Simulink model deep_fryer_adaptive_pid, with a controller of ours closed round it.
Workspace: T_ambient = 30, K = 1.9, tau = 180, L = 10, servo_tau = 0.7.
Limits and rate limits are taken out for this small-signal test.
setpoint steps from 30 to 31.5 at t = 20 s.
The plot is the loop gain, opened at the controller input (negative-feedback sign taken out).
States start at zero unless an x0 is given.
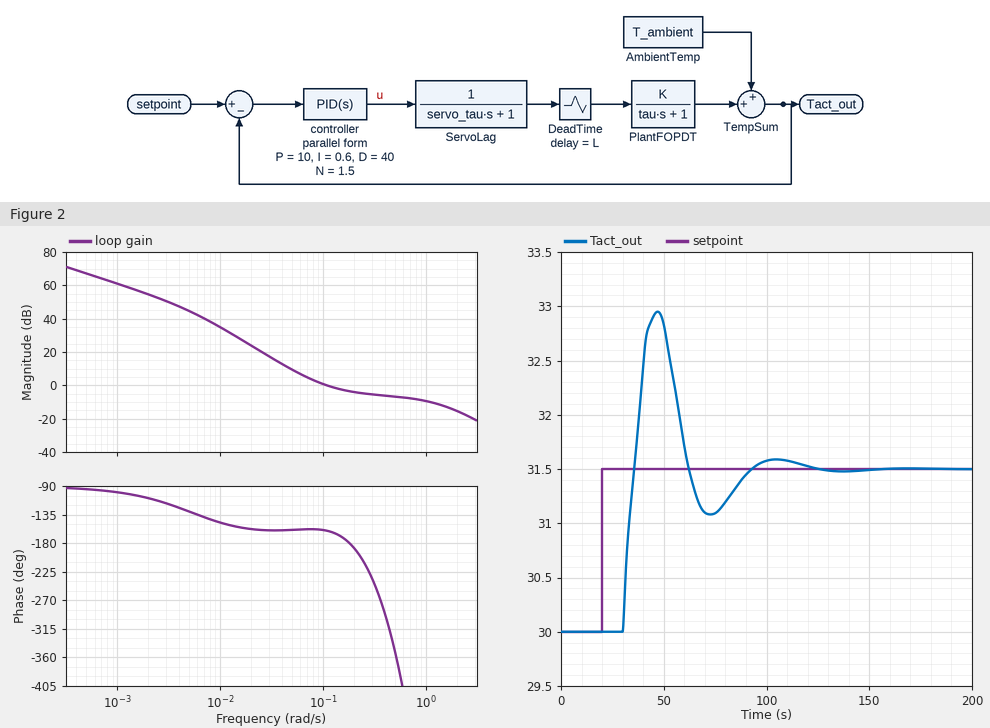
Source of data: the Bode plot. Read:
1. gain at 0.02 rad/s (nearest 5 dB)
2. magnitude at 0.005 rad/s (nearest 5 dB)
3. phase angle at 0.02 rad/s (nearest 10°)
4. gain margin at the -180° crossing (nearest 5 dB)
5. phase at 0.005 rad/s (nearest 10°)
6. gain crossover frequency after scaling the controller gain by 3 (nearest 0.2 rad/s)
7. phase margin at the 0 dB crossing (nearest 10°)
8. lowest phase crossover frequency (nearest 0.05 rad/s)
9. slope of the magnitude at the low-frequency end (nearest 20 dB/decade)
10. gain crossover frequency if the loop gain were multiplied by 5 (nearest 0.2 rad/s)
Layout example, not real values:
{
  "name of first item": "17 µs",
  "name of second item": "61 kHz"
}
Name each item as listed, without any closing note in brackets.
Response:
{
  "gain at 0.02 rad/s": "25 dB",
  "magnitude at 0.005 rad/s": "45 dB",
  "phase angle at 0.02 rad/s": "-160°",
  "gain margin at the -180° crossing": "5 dB",
  "phase at 0.005 rad/s": "-130°",
  "gain crossover frequency after scaling the controller gain by 3": "1.0 rad/s",
  "phase margin at the 0 dB crossing": "20°",
  "lowest phase crossover frequency": "0.20 rad/s",
  "slope of the magnitude at the low-frequency end": "-20 dB/decade",
  "gain crossover frequency if the loop gain were multiplied by 5": "1.8 rad/s"
}
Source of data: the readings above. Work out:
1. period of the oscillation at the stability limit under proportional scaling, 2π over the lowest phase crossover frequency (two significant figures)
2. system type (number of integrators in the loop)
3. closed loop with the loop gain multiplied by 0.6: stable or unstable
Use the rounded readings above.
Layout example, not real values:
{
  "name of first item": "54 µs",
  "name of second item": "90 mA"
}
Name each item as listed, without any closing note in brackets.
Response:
{
  "period of the oscillation at the stability limit under proportional scaling, 2π over the lowest phase crossover frequency": "31 s",
  "system type": "1",
  "closed loop with the loop gain multiplied by 0.6: stable or unstable": "stable"
}
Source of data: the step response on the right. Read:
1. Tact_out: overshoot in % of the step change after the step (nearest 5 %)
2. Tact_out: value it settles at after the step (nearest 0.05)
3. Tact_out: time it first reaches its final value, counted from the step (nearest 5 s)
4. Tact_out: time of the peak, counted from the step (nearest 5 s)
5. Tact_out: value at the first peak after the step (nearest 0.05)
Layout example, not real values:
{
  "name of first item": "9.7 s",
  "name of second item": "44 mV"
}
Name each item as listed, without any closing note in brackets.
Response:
{
  "Tact_out: overshoot in % of the step change after the step": "95 %",
  "Tact_out: value it settles at after the step": "31.50",
  "Tact_out: time it first reaches its final value, counted from the step": "15 s",
  "Tact_out: time of the peak, counted from the step": "25 s",
  "Tact_out: value at the first peak after the step": "32.95"
}
